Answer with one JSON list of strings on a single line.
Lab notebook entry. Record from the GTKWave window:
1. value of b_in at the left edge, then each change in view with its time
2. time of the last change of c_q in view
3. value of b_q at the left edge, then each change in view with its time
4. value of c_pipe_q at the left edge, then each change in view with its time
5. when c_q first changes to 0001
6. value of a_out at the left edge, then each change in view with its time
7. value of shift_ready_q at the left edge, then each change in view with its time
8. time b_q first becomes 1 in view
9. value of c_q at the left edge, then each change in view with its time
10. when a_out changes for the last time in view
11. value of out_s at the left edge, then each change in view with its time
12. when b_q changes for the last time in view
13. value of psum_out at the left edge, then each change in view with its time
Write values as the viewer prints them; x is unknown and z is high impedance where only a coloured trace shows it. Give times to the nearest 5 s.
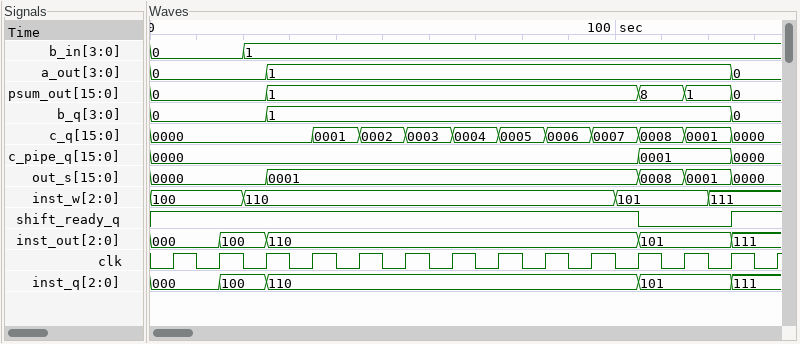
["0, 1 at 20 s", "125 s", "0, 1 at 25 s, 0 at 125 s", "0000, 0001 at 105 s, 0000 at 125 s", "35 s", "0, 1 at 25 s, 0 at 125 s", "1, 0 at 105 s, 1 at 125 s", "25 s", "0000, 0001 at 35 s, 0002 at 45 s, 0003 at 55 s, 0004 at 65 s, 0005 at 75 s, 0006 at 85 s, 0007 at 95 s, 0008 at 105 s, 0001 at 115 s, 0000 at 125 s", "125 s", "0000, 0001 at 25 s, 0008 at 105 s, 0001 at 115 s, 0000 at 125 s", "125 s", "0, 1 at 25 s, 8 at 105 s, 1 at 115 s, 0 at 125 s"]
